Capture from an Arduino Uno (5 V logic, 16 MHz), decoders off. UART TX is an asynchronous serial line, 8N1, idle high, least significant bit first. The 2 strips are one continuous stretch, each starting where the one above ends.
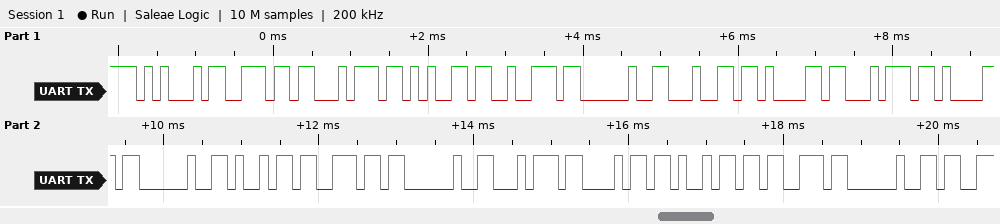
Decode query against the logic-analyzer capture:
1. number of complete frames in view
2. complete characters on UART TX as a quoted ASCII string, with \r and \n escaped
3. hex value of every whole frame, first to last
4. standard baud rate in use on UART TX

19
"Enter data in this "
45 6E 74 65 72 20 64 61 74 61 20 69 6E 20 74 68 69 73 20
9600 baud
